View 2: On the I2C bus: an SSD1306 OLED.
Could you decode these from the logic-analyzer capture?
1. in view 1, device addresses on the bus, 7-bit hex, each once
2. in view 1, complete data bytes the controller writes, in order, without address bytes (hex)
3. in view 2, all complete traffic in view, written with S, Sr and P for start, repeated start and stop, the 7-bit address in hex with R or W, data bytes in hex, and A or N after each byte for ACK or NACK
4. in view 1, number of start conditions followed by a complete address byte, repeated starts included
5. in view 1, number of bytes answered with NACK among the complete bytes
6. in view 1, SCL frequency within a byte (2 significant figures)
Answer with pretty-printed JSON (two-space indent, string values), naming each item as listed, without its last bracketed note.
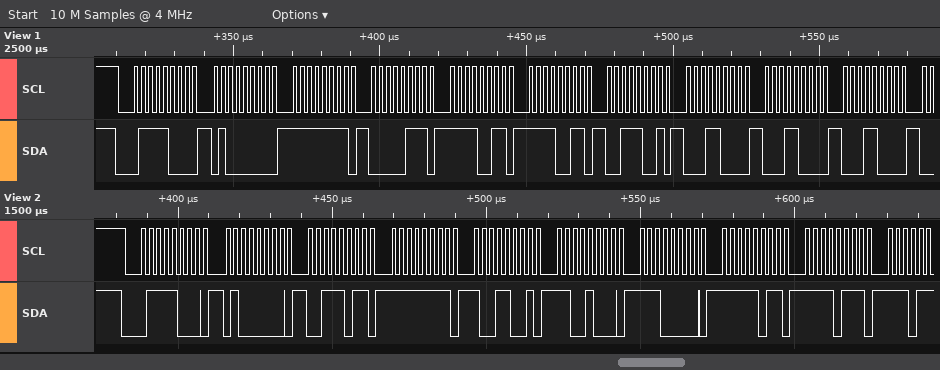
{
  "in view 1, device addresses on the bus, 7-bit hex, each once": "0x3C",
  "in view 1, complete data bytes the controller writes, in order, without address bytes": "40 FF 07 F3 F3 39 18 18 18",
  "in view 2, all complete traffic in view, written with S, Sr and P for start, repeated start and stop, the 7-bit address in hex with R or W, data bytes in hex, and A or N after each byte for ACK or NACK": "S 3CW A 40 A 3B A FF A 99 A C8 A E0 A FB A F7 A",
  "in view 1, number of start conditions followed by a complete address byte, repeated starts included": "1",
  "in view 1, number of bytes answered with NACK among the complete bytes": "0",
  "in view 1, SCL frequency within a byte": "400 kHz"
}
